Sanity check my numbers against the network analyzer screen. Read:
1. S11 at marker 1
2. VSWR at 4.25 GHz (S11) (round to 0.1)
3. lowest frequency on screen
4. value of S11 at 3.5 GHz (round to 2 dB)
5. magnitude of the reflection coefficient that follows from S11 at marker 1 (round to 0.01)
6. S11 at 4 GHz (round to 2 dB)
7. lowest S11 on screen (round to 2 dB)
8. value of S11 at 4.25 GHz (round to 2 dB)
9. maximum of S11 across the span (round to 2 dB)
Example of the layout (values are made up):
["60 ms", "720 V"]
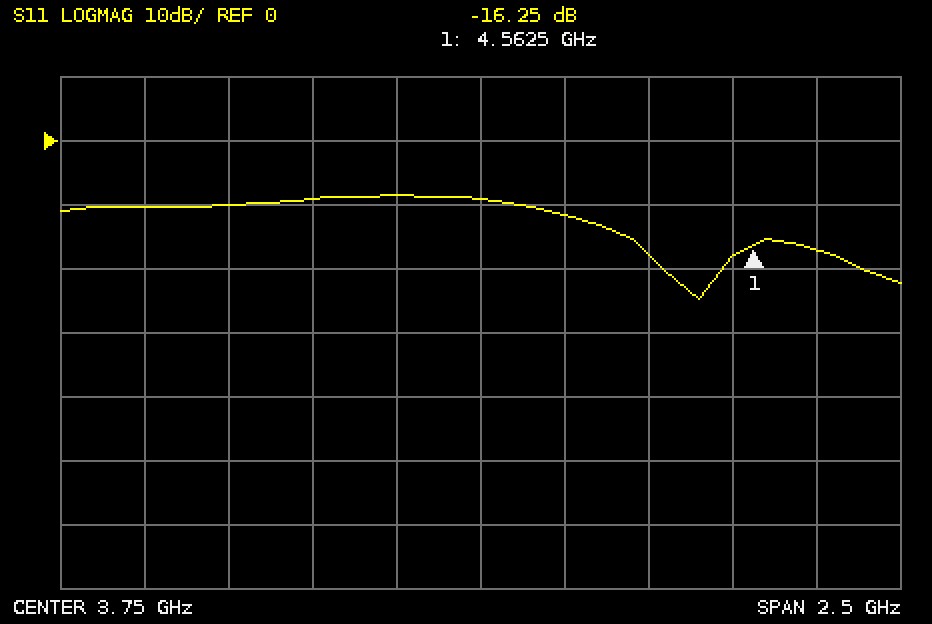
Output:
["-16.25 dB", "1.3", "2.5 GHz", "-8 dB", "0.15", "-12 dB", "-24 dB", "-18 dB", "-8 dB"]
